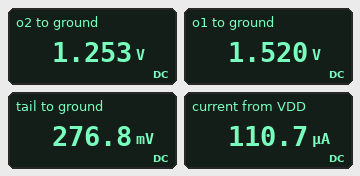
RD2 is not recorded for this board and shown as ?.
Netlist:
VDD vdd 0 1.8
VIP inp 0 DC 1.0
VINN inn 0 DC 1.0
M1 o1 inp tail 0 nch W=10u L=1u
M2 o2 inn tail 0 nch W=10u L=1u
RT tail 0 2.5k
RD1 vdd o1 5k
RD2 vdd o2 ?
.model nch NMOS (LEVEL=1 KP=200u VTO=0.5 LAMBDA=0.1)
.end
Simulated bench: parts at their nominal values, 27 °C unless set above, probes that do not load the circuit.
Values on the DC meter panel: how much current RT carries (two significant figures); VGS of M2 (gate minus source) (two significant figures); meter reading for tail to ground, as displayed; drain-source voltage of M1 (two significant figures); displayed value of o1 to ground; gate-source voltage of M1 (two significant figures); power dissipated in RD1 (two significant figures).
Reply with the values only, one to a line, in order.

110 µA
720 mV
276.8 mV
1.2 V
1.520 V
720 mV
16 µW
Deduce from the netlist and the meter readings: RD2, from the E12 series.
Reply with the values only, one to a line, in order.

10 kΩ
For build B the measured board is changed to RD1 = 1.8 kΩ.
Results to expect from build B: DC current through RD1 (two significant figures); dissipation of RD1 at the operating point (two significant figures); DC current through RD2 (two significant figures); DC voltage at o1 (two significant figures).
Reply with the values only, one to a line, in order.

57 µA
5.8 µW
54 µA
1.7 V
